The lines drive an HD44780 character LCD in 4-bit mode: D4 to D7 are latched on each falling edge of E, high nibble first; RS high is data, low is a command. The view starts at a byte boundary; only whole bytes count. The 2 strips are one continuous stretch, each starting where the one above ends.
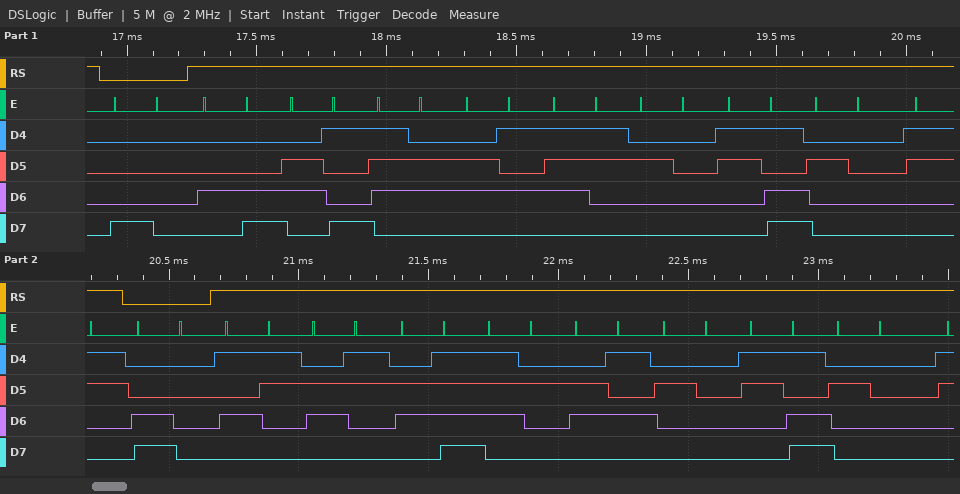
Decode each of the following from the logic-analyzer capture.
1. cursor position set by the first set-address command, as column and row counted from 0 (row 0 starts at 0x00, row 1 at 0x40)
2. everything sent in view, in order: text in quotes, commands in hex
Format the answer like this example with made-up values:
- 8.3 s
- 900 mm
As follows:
- column 0, row 0
- 0x80 "Lives = 3" 0xC0 "Score = "
